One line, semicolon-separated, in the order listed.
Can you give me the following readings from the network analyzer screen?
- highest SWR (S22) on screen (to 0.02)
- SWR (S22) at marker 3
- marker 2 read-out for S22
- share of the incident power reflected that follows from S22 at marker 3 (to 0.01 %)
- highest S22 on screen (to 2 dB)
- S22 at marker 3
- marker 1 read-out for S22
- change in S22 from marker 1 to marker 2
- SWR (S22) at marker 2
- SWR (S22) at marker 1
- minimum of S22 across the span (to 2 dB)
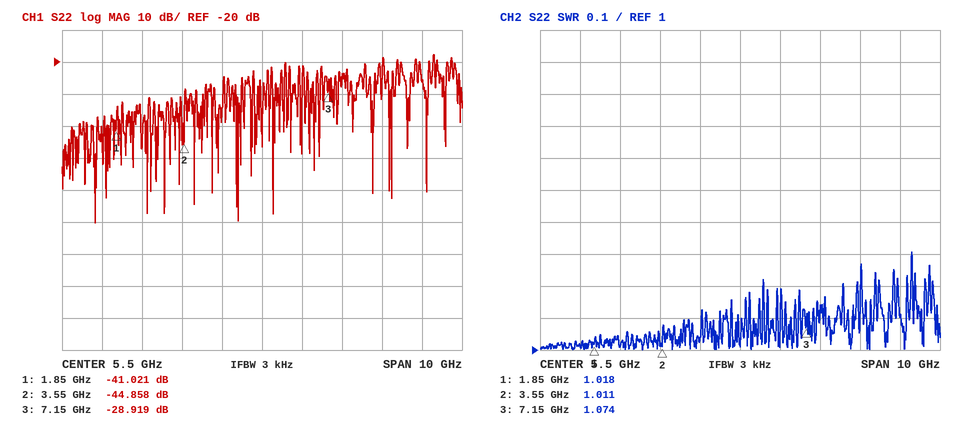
1.30; 1.074; -44.858 dB; 0.13 %; -18 dB; -28.919 dB; -41.021 dB; -3.837 dB; 1.011; 1.018; -70 dB
